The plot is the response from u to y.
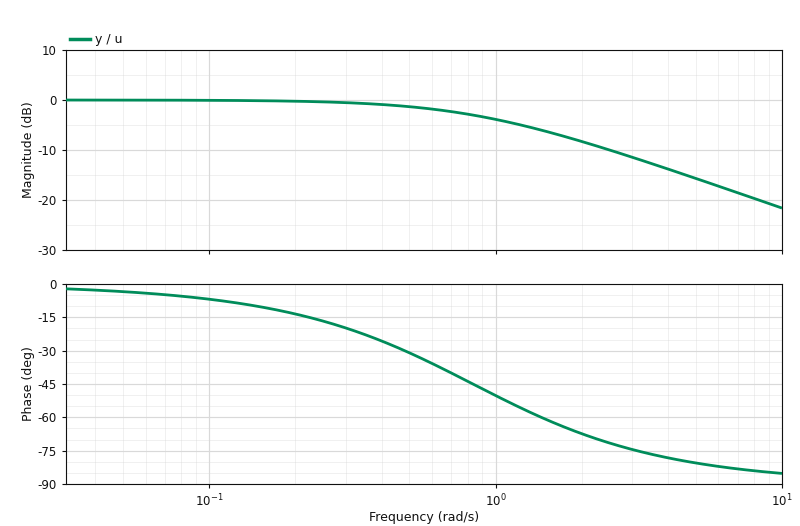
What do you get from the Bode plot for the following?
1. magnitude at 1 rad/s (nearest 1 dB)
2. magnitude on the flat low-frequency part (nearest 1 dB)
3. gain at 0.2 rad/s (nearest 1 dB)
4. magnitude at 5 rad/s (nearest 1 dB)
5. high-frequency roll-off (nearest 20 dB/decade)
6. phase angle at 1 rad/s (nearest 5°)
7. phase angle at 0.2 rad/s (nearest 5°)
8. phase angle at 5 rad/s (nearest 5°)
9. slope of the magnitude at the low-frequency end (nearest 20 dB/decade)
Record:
-4 dB
0 dB
0 dB
-16 dB
-20 dB/decade
-50°
-15°
-80°
0 dB/decade
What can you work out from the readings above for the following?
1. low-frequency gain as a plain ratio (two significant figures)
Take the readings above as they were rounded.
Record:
1.0
